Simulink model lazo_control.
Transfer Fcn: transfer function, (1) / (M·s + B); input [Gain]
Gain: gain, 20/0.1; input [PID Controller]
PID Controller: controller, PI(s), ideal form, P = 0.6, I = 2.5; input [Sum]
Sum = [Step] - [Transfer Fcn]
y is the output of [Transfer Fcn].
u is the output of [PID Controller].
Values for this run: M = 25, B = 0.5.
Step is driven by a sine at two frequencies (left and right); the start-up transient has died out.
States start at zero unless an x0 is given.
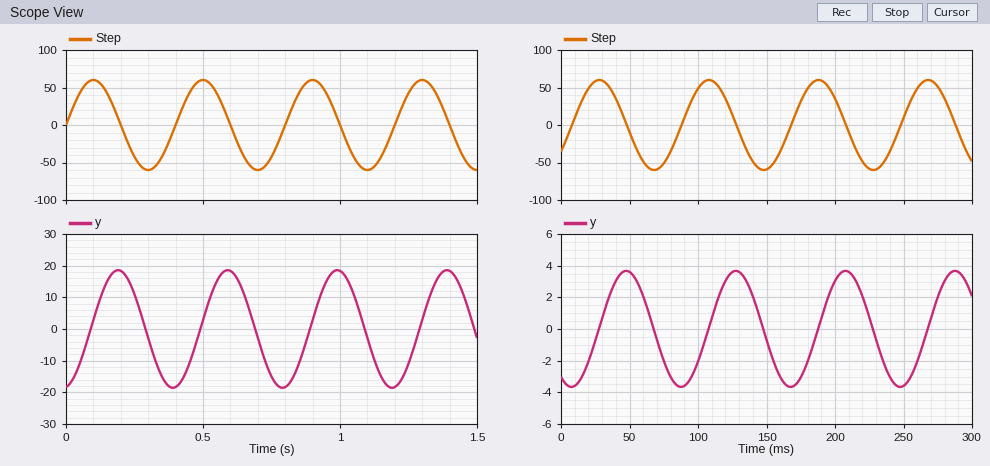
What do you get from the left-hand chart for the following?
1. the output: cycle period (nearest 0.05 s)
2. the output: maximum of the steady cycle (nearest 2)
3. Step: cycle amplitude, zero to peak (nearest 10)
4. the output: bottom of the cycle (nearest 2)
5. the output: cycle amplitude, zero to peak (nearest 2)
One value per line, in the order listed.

0.40 s
18
60
-18
18
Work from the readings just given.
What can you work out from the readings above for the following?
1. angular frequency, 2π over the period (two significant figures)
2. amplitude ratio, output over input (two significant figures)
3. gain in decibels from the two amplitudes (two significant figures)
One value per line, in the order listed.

16 rad/s
0.30
-10 dB
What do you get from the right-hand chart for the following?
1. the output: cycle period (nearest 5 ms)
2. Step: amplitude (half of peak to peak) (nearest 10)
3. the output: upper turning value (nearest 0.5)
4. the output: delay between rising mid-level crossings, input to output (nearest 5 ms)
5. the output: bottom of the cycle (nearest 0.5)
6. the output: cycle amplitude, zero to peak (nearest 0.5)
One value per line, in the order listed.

80 ms
60
3.5
20 ms
-3.5
3.5
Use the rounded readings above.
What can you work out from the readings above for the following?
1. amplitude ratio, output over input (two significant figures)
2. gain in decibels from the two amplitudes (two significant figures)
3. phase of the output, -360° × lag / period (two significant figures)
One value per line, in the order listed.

0.058
-25 dB
-90°
